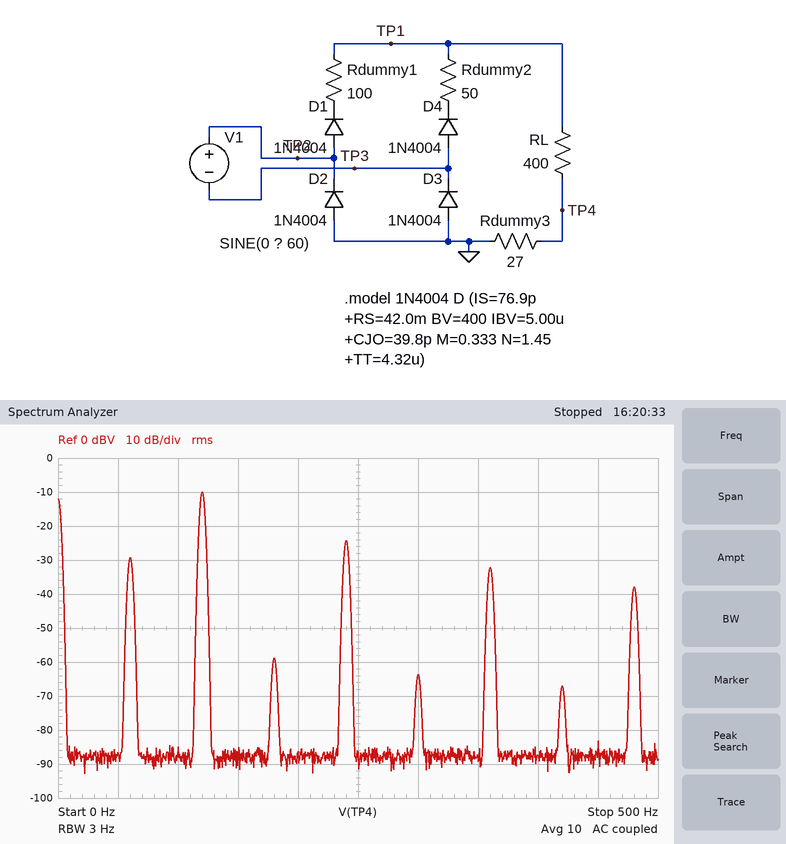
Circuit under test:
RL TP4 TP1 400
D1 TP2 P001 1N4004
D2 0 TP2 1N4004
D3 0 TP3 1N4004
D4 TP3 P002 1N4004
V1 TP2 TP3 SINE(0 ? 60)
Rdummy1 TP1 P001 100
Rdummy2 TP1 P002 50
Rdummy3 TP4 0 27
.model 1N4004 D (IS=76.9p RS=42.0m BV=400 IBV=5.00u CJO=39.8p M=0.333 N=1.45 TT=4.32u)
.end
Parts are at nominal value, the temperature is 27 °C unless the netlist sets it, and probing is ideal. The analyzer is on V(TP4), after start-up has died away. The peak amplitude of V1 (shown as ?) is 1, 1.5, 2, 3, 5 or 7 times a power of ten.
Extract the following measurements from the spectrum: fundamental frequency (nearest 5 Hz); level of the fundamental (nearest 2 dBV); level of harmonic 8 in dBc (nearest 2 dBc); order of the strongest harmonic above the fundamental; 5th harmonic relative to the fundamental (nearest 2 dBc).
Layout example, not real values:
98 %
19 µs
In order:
60 Hz
-30 dBV
-8 dBc
2
-34 dBc
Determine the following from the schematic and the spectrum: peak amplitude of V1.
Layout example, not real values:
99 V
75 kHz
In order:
20 V
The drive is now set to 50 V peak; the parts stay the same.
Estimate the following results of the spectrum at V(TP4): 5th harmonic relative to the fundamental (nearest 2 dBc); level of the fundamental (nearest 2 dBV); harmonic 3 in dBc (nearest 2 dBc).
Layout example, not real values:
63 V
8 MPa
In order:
-42 dBc
-20 dBV
-38 dBc
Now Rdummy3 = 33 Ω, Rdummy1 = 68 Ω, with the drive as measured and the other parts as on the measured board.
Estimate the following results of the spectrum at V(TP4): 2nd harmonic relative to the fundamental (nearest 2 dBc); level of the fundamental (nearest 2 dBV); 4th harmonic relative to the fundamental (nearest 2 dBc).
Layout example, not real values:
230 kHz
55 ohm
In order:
28 dBc
-36 dBV
14 dBc
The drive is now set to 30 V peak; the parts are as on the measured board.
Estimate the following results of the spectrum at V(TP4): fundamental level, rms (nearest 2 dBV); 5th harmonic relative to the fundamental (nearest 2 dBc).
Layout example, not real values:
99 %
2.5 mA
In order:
-26 dBV
-38 dBc
